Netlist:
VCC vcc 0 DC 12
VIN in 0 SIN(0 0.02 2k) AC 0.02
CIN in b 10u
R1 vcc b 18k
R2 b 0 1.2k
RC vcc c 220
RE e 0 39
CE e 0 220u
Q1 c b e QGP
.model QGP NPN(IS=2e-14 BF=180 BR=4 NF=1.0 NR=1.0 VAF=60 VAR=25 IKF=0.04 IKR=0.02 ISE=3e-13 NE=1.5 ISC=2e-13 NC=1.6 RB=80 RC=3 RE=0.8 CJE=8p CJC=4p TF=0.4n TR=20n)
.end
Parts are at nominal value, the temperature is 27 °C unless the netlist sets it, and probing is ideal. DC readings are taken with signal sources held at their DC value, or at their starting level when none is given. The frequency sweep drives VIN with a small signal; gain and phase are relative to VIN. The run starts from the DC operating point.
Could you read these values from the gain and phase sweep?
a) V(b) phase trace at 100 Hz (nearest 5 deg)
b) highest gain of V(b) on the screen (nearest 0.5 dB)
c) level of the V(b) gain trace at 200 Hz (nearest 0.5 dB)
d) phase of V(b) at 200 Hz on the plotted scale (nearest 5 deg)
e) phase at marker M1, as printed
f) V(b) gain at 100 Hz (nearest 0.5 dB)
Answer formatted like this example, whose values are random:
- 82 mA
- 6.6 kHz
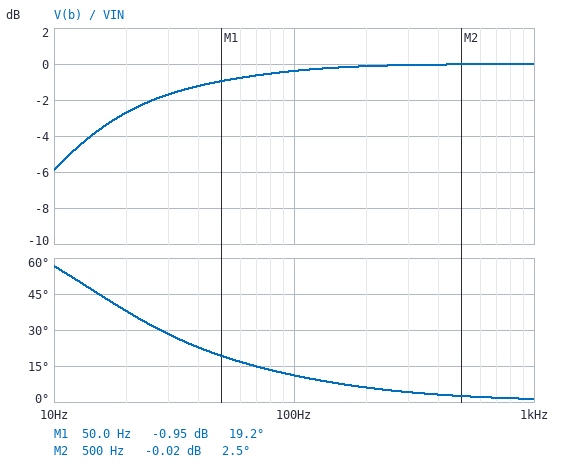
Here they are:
- 10 deg
- 0 dB
- 0 dB
- 5 deg
- 19.2 deg
- -0.5 dB
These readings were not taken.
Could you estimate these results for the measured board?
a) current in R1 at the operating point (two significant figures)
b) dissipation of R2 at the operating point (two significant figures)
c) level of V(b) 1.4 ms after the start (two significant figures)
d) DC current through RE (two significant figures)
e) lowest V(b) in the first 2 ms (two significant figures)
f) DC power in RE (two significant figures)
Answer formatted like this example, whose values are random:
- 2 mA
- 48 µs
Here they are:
- 630 µA
- 450 µW
- 710 mV
- 2.0 mA
- 710 mV
- 150 µW
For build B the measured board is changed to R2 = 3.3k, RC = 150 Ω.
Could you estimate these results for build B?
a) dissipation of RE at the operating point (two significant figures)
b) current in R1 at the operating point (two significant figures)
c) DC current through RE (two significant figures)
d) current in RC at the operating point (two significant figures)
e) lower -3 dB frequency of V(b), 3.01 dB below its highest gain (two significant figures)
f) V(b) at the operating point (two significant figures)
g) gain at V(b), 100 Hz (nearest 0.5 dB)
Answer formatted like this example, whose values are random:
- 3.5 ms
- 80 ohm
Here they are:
- 12 mW
- 590 µA
- 18 mA
- 17 mA
- 13 Hz
- 1.4 V
- -1.5 dB
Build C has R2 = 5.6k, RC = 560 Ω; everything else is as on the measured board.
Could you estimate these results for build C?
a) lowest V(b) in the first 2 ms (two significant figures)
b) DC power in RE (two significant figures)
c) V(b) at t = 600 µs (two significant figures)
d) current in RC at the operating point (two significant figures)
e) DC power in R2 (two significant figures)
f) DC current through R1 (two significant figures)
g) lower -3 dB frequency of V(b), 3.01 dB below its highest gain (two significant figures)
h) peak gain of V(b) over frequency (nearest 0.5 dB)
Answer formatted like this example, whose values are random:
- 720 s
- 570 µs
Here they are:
- 1.5 V
- 16 mW
- 1.6 V
- 20 mA
- 430 µW
- 580 µA
- 190 Hz
- 0 dB
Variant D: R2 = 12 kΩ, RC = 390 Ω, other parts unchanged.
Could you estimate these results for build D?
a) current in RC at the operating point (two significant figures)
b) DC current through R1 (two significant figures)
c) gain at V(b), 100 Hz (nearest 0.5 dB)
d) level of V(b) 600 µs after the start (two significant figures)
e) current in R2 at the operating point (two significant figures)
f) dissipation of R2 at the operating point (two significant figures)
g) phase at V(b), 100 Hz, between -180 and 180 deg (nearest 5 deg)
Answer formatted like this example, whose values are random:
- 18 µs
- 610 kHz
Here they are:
- 27 mA
- 560 µA
- -6.5 dB
- 1.9 V
- 160 µA
- 290 µW
- 55 deg
